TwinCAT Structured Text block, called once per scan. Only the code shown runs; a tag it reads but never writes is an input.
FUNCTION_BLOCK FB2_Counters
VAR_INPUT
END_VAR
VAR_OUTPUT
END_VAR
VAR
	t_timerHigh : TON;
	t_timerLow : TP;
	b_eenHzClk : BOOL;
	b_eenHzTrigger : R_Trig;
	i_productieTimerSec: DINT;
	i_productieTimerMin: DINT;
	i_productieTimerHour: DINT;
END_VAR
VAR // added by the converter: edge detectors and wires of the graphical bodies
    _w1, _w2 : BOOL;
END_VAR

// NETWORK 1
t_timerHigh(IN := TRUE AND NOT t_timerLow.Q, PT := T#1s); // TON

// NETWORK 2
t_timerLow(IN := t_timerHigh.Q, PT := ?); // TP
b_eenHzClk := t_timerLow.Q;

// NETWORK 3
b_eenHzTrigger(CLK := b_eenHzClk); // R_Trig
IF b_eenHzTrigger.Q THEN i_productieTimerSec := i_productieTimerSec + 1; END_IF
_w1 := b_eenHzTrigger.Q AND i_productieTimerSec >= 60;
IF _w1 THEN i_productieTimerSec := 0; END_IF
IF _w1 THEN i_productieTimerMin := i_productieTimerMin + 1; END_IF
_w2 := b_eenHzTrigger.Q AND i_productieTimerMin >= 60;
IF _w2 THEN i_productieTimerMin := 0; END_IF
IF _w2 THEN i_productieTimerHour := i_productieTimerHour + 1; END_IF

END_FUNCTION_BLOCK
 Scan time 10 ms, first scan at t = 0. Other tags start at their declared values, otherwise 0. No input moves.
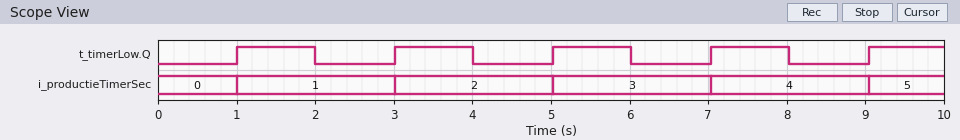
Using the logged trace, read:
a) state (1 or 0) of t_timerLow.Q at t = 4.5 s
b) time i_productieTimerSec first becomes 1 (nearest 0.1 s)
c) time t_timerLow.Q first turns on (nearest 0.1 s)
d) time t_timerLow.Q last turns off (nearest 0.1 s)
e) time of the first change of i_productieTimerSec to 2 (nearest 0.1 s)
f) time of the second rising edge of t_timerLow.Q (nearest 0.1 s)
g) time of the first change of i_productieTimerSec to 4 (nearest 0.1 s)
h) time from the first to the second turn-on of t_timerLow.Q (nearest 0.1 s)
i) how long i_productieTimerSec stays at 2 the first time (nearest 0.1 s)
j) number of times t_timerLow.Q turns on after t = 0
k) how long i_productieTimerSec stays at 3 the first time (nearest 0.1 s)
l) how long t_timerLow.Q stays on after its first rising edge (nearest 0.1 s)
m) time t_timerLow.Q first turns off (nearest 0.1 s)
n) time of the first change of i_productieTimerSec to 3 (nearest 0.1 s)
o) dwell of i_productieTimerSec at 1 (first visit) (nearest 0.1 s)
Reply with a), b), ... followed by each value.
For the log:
a) 0
b) 1.0 s
c) 1.0 s
d) 8.0 s
e) 3.0 s
f) 3.0 s
g) 7.0 s
h) 2.0 s
i) 2.0 s
j) 5
k) 2.0 s
l) 1.0 s
m) 2.0 s
n) 5.0 s
o) 2.0 s
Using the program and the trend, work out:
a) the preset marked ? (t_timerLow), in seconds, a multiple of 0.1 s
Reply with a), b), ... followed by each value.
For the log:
a) 1.0 s
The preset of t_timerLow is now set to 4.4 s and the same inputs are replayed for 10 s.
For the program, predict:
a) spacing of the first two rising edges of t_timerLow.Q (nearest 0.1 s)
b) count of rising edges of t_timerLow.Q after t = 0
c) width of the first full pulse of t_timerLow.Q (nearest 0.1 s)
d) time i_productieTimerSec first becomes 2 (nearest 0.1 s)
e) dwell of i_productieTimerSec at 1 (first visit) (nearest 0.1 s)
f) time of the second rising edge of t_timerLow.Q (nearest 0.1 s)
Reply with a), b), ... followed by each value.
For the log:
a) 5.4 s
b) 2
c) 4.4 s
d) 6.4 s
e) 5.4 s
f) 6.4 s
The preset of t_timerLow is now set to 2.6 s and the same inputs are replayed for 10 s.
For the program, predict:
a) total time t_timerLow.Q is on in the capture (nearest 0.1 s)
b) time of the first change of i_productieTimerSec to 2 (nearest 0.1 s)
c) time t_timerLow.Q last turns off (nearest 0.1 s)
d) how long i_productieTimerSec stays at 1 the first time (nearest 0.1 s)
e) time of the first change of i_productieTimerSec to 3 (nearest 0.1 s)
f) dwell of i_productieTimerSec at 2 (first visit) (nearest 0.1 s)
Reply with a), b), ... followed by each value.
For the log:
a) 7.0 s
b) 4.6 s
c) 7.2 s
d) 3.6 s
e) 8.2 s
f) 3.6 s
